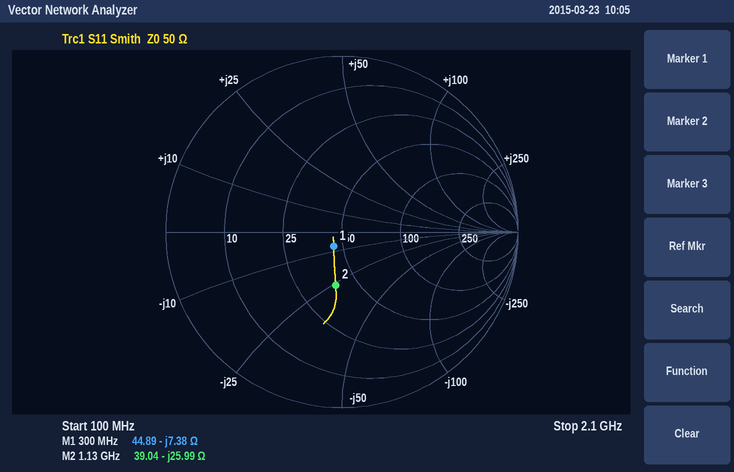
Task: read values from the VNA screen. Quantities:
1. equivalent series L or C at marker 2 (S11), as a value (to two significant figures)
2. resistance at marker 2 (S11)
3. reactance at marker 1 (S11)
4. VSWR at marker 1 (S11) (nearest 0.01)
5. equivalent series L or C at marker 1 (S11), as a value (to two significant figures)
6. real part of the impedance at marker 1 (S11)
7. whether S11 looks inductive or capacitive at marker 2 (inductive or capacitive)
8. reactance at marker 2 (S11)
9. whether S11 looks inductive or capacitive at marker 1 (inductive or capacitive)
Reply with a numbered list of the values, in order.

1. 5.4 pF
2. 39.04 Ω
3. -7.38 Ω
4. 1.21
5. 72 pF
6. 44.89 Ω
7. capacitive
8. -25.99 Ω
9. capacitive
